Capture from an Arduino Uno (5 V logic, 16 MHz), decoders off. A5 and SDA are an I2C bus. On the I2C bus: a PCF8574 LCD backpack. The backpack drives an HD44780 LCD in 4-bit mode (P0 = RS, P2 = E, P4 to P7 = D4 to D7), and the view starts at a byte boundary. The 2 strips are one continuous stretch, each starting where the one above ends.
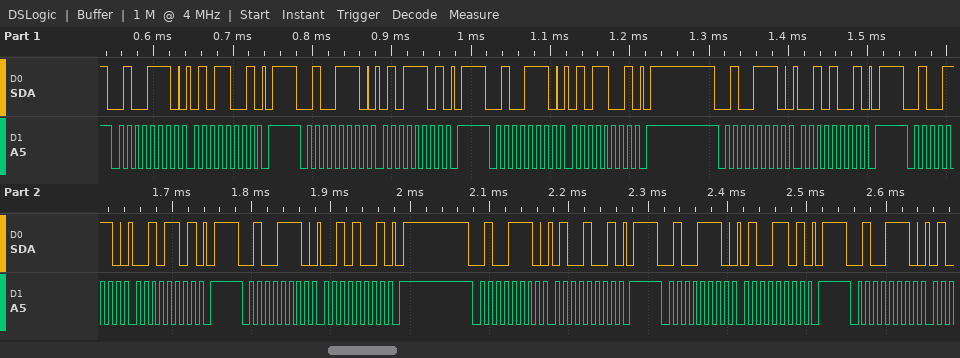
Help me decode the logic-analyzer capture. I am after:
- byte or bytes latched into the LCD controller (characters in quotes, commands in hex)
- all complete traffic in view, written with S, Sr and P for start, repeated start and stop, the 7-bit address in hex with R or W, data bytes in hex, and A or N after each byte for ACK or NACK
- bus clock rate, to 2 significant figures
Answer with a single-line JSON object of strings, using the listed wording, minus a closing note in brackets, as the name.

{"byte or bytes latched into the LCD controller": "'R'", "all complete traffic in view, written with S, Sr and P for start, repeated start and stop, the 7-bit address in hex with R or W, data bytes in hex, and A or N after each byte for ACK or NACK": "S 27W A 59 A P S 27W A 5D A P S 27W A 59 A P S 27W A 29 A P S 27W A 2D A P S 27W A 29 A P S 27W A 49 A P S 27W A 4D A P S 27W A", "bus clock rate, to 2 significant figures": "100 kHz"}
